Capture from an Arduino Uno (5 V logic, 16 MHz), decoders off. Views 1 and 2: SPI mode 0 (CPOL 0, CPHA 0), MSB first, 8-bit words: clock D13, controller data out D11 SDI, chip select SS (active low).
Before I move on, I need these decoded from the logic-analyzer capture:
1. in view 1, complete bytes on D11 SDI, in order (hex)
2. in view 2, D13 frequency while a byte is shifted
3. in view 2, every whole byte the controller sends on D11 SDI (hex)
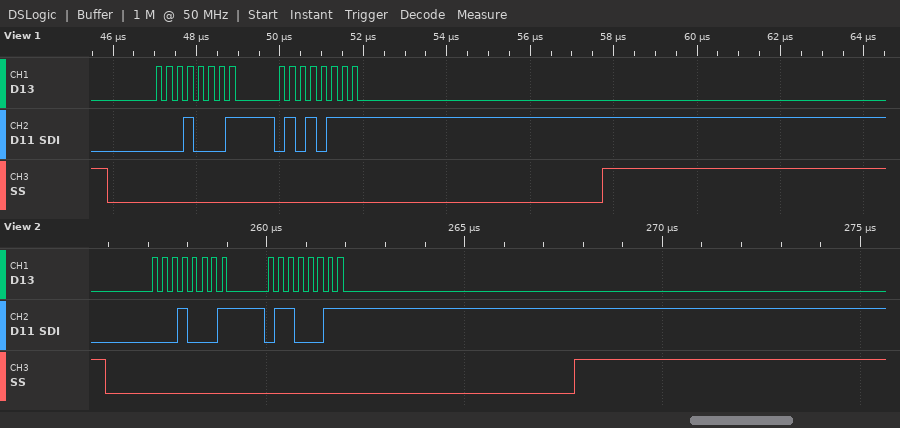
11 57
4 MHz
11 63
